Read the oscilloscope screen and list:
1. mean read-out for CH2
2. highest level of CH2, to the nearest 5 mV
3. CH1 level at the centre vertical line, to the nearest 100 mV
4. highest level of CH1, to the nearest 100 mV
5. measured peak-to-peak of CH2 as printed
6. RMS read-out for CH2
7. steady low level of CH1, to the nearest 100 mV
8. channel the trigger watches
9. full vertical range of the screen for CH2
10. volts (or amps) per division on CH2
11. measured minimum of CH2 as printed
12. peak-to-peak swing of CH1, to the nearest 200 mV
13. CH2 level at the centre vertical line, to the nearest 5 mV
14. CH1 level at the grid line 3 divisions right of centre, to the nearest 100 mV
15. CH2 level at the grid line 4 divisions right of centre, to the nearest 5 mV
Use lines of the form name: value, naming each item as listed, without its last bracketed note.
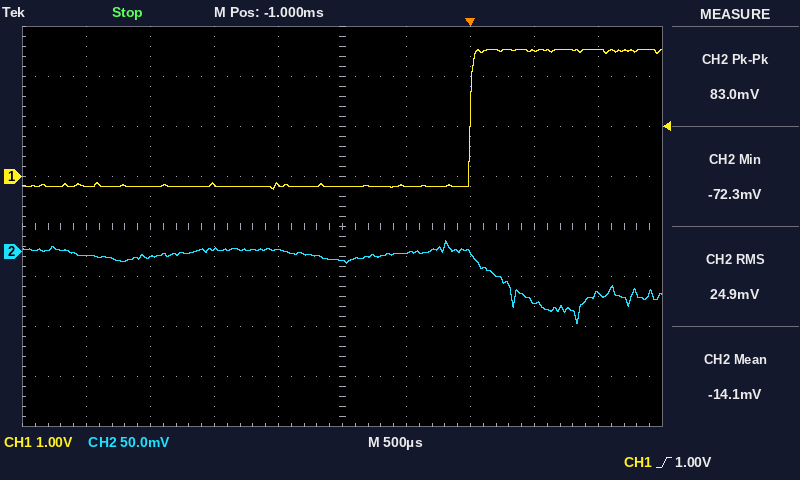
mean read-out for CH2: -14.1 mV
highest level of CH2, to the nearest 5 mV: 10 mV
CH1 level at the centre vertical line, to the nearest 100 mV: -200 mV
highest level of CH1, to the nearest 100 mV: 2.5 V
measured peak-to-peak of CH2 as printed: 83.0 mV
RMS read-out for CH2: 24.9 mV
steady low level of CH1, to the nearest 100 mV: -200 mV
channel the trigger watches: CH1
full vertical range of the screen for CH2: 400 mV
volts (or amps) per division on CH2: 50 mV
measured minimum of CH2 as printed: -72.3 mV
peak-to-peak swing of CH1, to the nearest 200 mV: 2.8 V
CH2 level at the centre vertical line, to the nearest 5 mV: -10 mV
CH1 level at the grid line 3 divisions right of centre, to the nearest 100 mV: 2.5 V
CH2 level at the grid line 4 divisions right of centre, to the nearest 5 mV: -40 mV
